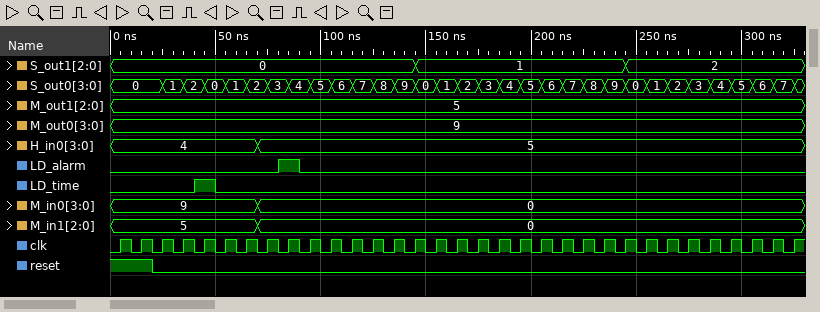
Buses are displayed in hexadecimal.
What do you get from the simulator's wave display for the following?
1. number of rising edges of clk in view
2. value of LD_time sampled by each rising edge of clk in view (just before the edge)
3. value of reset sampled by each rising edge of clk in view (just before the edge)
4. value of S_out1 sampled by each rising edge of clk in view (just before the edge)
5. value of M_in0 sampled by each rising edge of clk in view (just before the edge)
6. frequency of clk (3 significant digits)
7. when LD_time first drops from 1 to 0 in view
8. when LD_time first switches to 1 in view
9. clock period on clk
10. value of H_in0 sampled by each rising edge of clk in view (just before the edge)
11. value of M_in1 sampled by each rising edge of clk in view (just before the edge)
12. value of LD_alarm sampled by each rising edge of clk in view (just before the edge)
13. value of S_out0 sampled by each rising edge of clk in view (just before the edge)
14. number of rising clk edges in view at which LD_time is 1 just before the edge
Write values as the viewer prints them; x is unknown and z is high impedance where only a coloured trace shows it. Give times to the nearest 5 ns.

33
0 0 0 0 1 0 0 0 0 0 0 0 0 0 0 0 0 0 0 0 0 0 0 0 0 0 0 0 0 0 0 0 0
1 1 0 0 0 0 0 0 0 0 0 0 0 0 0 0 0 0 0 0 0 0 0 0 0 0 0 0 0 0 0 0 0
0, 0, 0, 0, 0, 0, 0, 0, 0, 0, 0, 0, 0, 0, 0, 1, 1, 1, 1, 1, 1, 1, 1, 1, 1, 2, 2, 2, 2, 2, 2, 2, 2
9, 9, 9, 9, 9, 9, 9, 0, 0, 0, 0, 0, 0, 0, 0, 0, 0, 0, 0, 0, 0, 0, 0, 0, 0, 0, 0, 0, 0, 0, 0, 0, 0
100 MHz
50 ns
40 ns
10 ns
4, 4, 4, 4, 4, 4, 4, 5, 5, 5, 5, 5, 5, 5, 5, 5, 5, 5, 5, 5, 5, 5, 5, 5, 5, 5, 5, 5, 5, 5, 5, 5, 5
5, 5, 5, 5, 5, 5, 5, 0, 0, 0, 0, 0, 0, 0, 0, 0, 0, 0, 0, 0, 0, 0, 0, 0, 0, 0, 0, 0, 0, 0, 0, 0, 0
0 0 0 0 0 0 0 0 1 0 0 0 0 0 0 0 0 0 0 0 0 0 0 0 0 0 0 0 0 0 0 0 0
0, 0, 0, 1, 2, 0, 1, 2, 3, 4, 5, 6, 7, 8, 9, 0, 1, 2, 3, 4, 5, 6, 7, 8, 9, 0, 1, 2, 3, 4, 5, 6, 7
1
